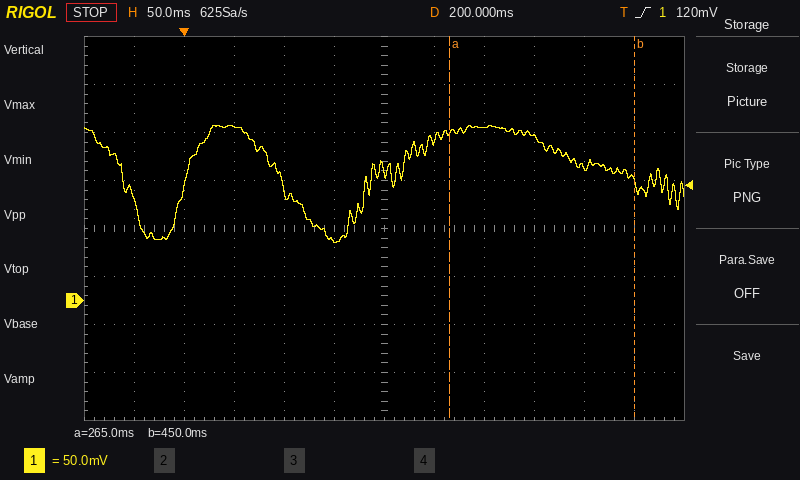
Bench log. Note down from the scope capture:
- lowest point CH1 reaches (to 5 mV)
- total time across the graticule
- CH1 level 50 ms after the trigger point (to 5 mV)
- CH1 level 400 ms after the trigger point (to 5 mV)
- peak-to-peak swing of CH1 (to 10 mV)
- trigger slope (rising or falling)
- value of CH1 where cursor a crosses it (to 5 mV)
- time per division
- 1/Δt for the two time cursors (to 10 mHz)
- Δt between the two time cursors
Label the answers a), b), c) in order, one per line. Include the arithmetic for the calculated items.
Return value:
a) 60 mV
b) 600 ms
c) 180 mV
d) 140 mV
e) 120 mV
f) rising
g) 175 mV
h) 50 ms
i) 1 / 185 ms ≈ 5.41 Hz
j) 450 ms − (265 ms) = 185 ms
